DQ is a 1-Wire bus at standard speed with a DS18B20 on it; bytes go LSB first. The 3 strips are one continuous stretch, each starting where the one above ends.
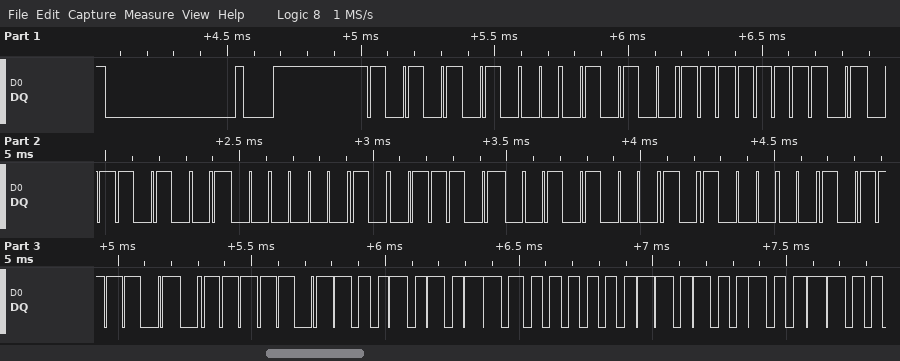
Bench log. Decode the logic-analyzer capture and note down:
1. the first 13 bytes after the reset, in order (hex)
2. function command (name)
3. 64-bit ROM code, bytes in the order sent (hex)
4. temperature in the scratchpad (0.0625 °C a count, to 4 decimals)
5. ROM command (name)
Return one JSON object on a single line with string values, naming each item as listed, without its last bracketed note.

{"the first 13 bytes after the reset, in order": "55 28 FF 5A 02 B9 14 05 BD BE A9 01 4B", "function command": "Read Scratchpad", "64-bit ROM code, bytes in the order sent": "28 FF 5A 02 B9 14 05 BD", "temperature in the scratchpad": "26.5625 °C", "ROM command": "Match ROM"}
